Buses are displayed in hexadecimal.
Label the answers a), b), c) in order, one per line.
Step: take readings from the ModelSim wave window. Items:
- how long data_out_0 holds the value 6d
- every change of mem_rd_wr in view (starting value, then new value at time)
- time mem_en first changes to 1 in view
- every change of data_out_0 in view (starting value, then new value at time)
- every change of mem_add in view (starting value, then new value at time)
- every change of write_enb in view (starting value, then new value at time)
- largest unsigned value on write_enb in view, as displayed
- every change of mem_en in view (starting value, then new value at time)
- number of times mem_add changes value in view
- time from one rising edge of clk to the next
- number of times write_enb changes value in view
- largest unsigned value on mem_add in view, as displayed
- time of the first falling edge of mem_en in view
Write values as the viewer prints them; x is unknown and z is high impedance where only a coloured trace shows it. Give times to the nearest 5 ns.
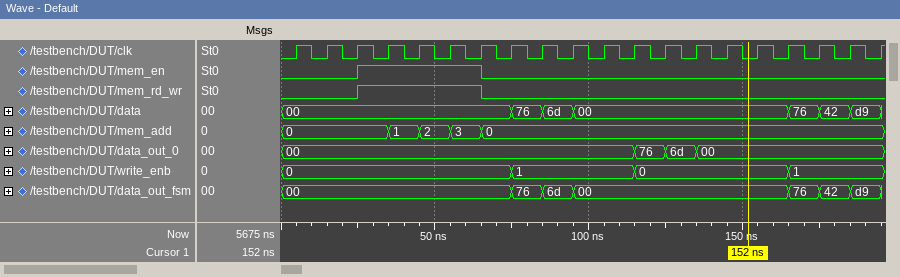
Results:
a) 10 ns
b) 0, 1 at 25 ns, 0 at 65 ns
c) 25 ns
d) 00, 76 at 115 ns, 6d at 125 ns, 00 at 135 ns
e) 0, 1 at 35 ns, 2 at 45 ns, 3 at 55 ns, 0 at 65 ns
f) 0, 1 at 75 ns, 0 at 115 ns, 1 at 165 ns
g) 1
h) 0, 1 at 25 ns, 0 at 65 ns
i) 4
j) 10 ns
k) 3
l) 3
m) 65 ns
